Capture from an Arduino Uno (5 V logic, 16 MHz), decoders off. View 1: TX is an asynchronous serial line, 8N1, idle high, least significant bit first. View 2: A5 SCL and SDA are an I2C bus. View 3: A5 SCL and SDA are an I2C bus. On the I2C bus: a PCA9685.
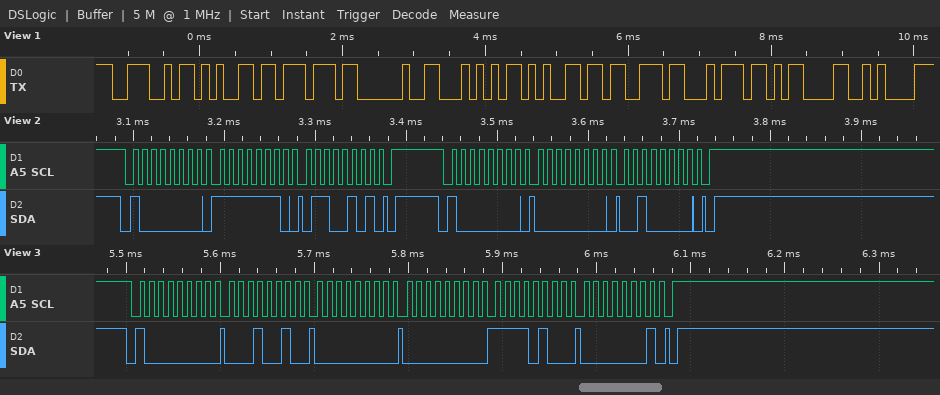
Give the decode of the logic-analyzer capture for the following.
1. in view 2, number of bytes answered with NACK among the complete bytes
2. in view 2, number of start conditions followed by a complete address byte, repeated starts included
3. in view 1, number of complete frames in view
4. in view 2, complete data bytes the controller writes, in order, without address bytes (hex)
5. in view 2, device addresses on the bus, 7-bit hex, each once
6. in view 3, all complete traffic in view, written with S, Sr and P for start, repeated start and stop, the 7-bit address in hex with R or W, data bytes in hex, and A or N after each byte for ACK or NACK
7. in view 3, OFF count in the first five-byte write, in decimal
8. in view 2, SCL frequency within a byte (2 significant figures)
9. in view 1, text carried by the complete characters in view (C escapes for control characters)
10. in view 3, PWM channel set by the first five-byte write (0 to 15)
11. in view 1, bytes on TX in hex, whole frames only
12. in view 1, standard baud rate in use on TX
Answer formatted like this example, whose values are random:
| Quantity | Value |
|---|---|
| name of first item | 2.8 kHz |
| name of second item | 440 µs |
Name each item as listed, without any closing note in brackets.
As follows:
| Quantity | Value |
|---|---|
| in view 2, number of bytes answered with NACK among the complete bytes | 0 |
| in view 2, number of start conditions followed by a complete address byte, repeated starts included | 2 |
| in view 1, number of complete frames in view | 10 |
| in view 2, complete data bytes the controller writes, in order, without address bytes | FE 65 00 20 |
| in view 2, device addresses on the bus, 7-bit hex, each once | 0x40 |
| in view 3, all complete traffic in view, written with S, Sr and P for start, repeated start and stop, the 7-bit address in hex with R or W, data bytes in hex, and A or N after each byte for ACK or NACK | S 40W A 12 A 00 A 00 A F4 A 01 A P |
| in view 3, OFF count in the first five-byte write, in decimal | 500 |
| in view 2, SCL frequency within a byte | 100 kHz |
| in view 1, text carried by the complete characters in view | "New Test\r\n" |
| in view 3, PWM channel set by the first five-byte write | 3 |
| in view 1, bytes on TX in hex, whole frames only | 4E 65 77 20 54 65 73 74 0D 0A |
| in view 1, standard baud rate in use on TX | 9600 baud |
